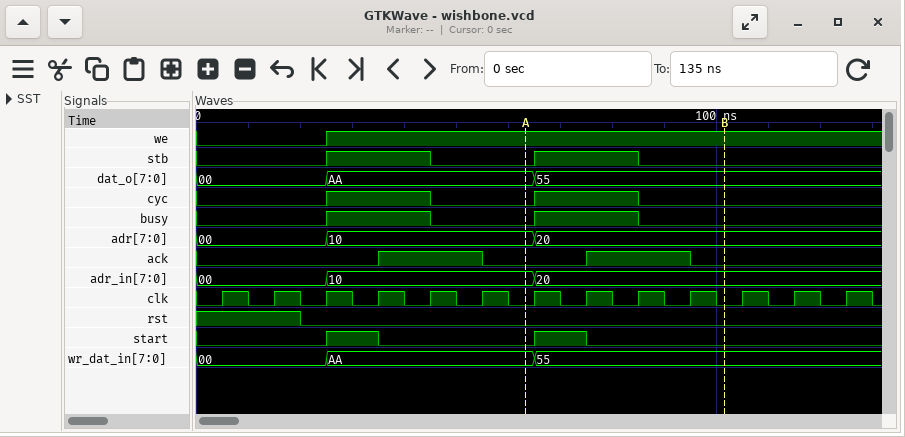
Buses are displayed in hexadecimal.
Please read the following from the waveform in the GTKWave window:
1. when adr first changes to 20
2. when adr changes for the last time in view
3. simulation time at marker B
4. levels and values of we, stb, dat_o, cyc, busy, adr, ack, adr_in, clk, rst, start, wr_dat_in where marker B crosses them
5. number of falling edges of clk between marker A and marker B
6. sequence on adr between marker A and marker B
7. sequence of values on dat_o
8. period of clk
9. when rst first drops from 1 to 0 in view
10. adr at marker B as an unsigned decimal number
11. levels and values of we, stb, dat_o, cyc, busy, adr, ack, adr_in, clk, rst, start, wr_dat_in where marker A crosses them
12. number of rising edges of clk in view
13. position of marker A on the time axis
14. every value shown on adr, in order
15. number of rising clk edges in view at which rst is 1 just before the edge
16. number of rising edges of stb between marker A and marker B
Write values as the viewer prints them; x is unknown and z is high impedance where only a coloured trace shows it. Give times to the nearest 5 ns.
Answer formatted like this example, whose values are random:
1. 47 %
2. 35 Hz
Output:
1. 65 ns
2. 65 ns
3. 100 ns
4. we=1, stb=0, dat_o=55, cyc=0, busy=0, adr=20, ack=0, adr_in=20, clk=0, rst=0, start=0, wr_dat_in=55
5. 4
6. 10, 20
7. 00, AA, 55
8. 10 ns
9. 20 ns
10. 32
11. we=1, stb=0, dat_o=AA, cyc=0, busy=0, adr=10, ack=0, adr_in=10, clk=0, rst=0, start=0, wr_dat_in=AA
12. 13
13. 65 ns
14. 00, 10, 20
15. 2
16. 1
